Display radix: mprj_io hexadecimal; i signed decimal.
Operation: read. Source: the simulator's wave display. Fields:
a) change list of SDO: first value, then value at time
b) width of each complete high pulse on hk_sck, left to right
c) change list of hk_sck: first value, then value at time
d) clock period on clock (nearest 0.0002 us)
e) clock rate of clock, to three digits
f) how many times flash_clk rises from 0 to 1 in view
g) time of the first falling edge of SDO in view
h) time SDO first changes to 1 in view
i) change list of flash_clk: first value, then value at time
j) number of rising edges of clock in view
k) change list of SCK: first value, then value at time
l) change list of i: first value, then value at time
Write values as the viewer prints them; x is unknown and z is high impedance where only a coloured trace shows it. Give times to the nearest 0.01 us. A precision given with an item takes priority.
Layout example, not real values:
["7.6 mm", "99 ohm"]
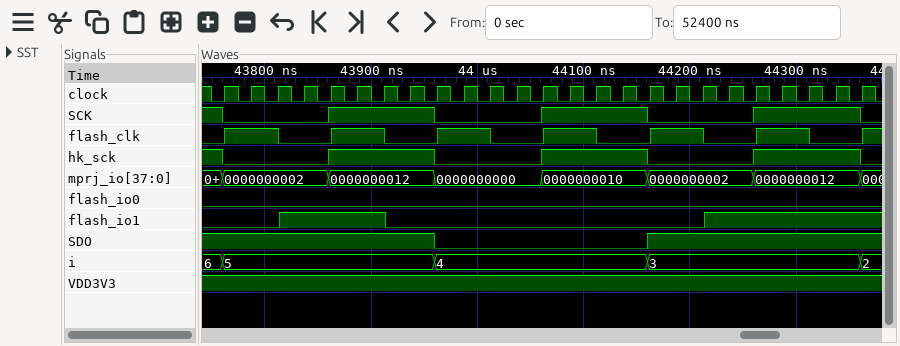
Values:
["1, 0 at 43.96 us, 1 at 44.16 us", "0.1 us, 0.1 us, 0.1 us", "1, 0 at 43.76 us, 1 at 43.86 us, 0 at 43.96 us, 1 at 44.06 us, 0 at 44.16 us, 1 at 44.26 us, 0 at 44.36 us", "0.025 us", "40.0 MHz", "7", "43.96 us", "44.16 us", "0, 1 at 43.76 us, 0 at 43.81 us, 1 at 43.86 us, 0 at 43.91 us, 1 at 43.96 us, 0 at 44.01 us, 1 at 44.06 us, 0 at 44.11 us, 1 at 44.16 us, 0 at 44.21 us, 1 at 44.26 us, 0 at 44.31 us, 1 at 44.36 us", "25", "1, 0 at 43.76 us, 1 at 43.86 us, 0 at 43.96 us, 1 at 44.06 us, 0 at 44.16 us, 1 at 44.26 us, 0 at 44.36 us", "6, 5 at 43.76 us, 4 at 43.96 us, 3 at 44.16 us, 2 at 44.36 us"]
